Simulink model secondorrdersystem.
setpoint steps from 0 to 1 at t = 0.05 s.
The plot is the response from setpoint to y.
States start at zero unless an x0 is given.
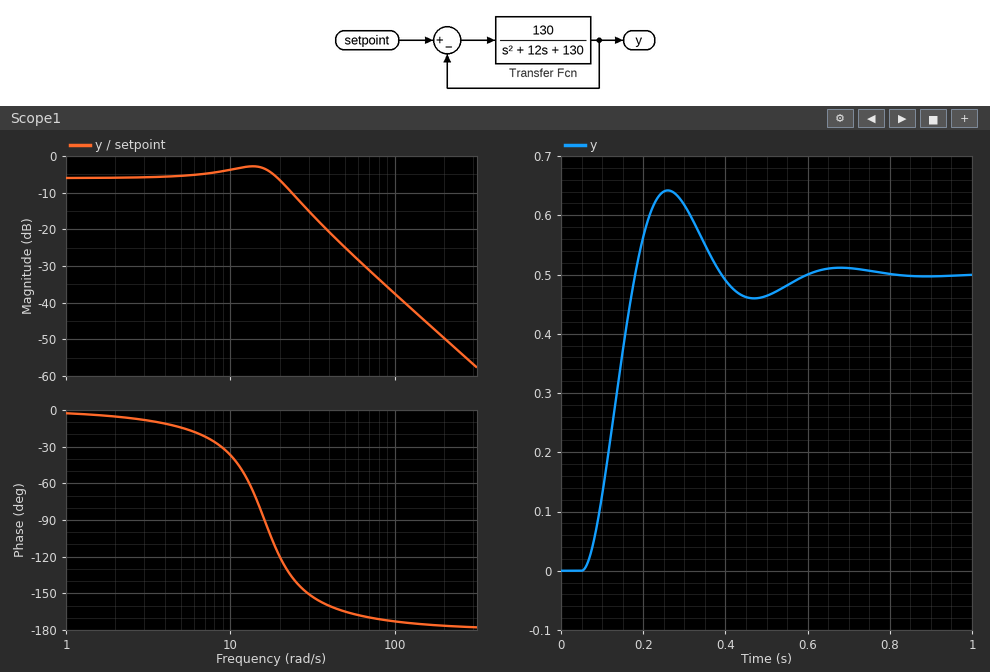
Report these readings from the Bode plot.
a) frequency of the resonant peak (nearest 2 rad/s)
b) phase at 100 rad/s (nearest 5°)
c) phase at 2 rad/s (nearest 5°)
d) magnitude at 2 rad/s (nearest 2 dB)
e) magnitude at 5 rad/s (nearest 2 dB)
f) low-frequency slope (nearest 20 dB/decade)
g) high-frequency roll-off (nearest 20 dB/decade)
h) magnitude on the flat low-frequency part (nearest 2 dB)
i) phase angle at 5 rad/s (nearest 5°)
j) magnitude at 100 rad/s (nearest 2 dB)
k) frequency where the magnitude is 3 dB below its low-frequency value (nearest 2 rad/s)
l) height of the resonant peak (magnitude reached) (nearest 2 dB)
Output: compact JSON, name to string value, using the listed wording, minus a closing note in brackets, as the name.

{"frequency of the resonant peak": "14 rad/s", "phase at 100 rad/s": "-175°", "phase at 2 rad/s": "-5°", "magnitude at 2 rad/s": "-6 dB", "magnitude at 5 rad/s": "-6 dB", "low-frequency slope": "0 dB/decade", "high-frequency roll-off": "-40 dB/decade", "magnitude on the flat low-frequency part": "-6 dB", "phase angle at 5 rad/s": "-15°", "magnitude at 100 rad/s": "-38 dB", "frequency where the magnitude is 3 dB below its low-frequency value": "22 rad/s", "height of the resonant peak (magnitude reached)": "-2 dB"}
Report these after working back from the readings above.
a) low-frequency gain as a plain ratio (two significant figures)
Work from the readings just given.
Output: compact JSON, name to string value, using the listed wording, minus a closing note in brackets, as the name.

{"low-frequency gain as a plain ratio": "0.50"}
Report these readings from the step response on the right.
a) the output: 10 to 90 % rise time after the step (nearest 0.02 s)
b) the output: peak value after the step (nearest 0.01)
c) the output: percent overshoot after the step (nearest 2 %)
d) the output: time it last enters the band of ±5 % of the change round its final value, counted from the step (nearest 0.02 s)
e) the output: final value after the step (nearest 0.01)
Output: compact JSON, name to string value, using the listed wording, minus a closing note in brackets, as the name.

{"the output: 10 to 90 % rise time after the step": "0.08 s", "the output: peak value after the step": "0.64", "the output: percent overshoot after the step": "28 %", "the output: time it last enters the band of ±5 % of the change round its final value, counted from the step": "0.48 s", "the output: final value after the step": "0.50"}
